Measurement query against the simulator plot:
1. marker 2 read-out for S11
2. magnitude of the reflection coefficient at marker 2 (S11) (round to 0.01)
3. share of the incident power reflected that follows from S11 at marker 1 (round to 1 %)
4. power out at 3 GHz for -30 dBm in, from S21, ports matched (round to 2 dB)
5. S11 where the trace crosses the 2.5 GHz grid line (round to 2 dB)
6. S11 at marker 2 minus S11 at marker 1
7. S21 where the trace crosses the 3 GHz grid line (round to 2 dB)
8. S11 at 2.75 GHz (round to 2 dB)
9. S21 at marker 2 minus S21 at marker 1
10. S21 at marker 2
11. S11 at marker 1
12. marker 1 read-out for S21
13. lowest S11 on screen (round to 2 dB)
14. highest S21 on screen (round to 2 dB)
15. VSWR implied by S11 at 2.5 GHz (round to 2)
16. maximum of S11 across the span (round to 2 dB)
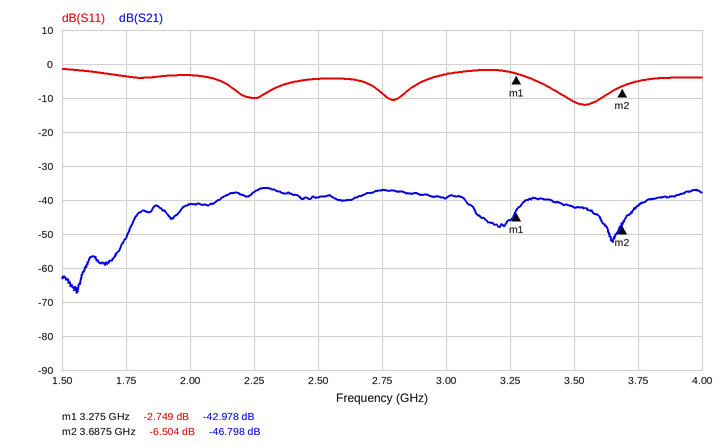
-6.504 dB
0.47
53 %
-70 dBm
-4 dB
-3.755 dB
-40 dB
-8 dB
-3.820 dB
-46.798 dB
-2.749 dB
-42.978 dB
-12 dB
-36 dB
4
-2 dB
